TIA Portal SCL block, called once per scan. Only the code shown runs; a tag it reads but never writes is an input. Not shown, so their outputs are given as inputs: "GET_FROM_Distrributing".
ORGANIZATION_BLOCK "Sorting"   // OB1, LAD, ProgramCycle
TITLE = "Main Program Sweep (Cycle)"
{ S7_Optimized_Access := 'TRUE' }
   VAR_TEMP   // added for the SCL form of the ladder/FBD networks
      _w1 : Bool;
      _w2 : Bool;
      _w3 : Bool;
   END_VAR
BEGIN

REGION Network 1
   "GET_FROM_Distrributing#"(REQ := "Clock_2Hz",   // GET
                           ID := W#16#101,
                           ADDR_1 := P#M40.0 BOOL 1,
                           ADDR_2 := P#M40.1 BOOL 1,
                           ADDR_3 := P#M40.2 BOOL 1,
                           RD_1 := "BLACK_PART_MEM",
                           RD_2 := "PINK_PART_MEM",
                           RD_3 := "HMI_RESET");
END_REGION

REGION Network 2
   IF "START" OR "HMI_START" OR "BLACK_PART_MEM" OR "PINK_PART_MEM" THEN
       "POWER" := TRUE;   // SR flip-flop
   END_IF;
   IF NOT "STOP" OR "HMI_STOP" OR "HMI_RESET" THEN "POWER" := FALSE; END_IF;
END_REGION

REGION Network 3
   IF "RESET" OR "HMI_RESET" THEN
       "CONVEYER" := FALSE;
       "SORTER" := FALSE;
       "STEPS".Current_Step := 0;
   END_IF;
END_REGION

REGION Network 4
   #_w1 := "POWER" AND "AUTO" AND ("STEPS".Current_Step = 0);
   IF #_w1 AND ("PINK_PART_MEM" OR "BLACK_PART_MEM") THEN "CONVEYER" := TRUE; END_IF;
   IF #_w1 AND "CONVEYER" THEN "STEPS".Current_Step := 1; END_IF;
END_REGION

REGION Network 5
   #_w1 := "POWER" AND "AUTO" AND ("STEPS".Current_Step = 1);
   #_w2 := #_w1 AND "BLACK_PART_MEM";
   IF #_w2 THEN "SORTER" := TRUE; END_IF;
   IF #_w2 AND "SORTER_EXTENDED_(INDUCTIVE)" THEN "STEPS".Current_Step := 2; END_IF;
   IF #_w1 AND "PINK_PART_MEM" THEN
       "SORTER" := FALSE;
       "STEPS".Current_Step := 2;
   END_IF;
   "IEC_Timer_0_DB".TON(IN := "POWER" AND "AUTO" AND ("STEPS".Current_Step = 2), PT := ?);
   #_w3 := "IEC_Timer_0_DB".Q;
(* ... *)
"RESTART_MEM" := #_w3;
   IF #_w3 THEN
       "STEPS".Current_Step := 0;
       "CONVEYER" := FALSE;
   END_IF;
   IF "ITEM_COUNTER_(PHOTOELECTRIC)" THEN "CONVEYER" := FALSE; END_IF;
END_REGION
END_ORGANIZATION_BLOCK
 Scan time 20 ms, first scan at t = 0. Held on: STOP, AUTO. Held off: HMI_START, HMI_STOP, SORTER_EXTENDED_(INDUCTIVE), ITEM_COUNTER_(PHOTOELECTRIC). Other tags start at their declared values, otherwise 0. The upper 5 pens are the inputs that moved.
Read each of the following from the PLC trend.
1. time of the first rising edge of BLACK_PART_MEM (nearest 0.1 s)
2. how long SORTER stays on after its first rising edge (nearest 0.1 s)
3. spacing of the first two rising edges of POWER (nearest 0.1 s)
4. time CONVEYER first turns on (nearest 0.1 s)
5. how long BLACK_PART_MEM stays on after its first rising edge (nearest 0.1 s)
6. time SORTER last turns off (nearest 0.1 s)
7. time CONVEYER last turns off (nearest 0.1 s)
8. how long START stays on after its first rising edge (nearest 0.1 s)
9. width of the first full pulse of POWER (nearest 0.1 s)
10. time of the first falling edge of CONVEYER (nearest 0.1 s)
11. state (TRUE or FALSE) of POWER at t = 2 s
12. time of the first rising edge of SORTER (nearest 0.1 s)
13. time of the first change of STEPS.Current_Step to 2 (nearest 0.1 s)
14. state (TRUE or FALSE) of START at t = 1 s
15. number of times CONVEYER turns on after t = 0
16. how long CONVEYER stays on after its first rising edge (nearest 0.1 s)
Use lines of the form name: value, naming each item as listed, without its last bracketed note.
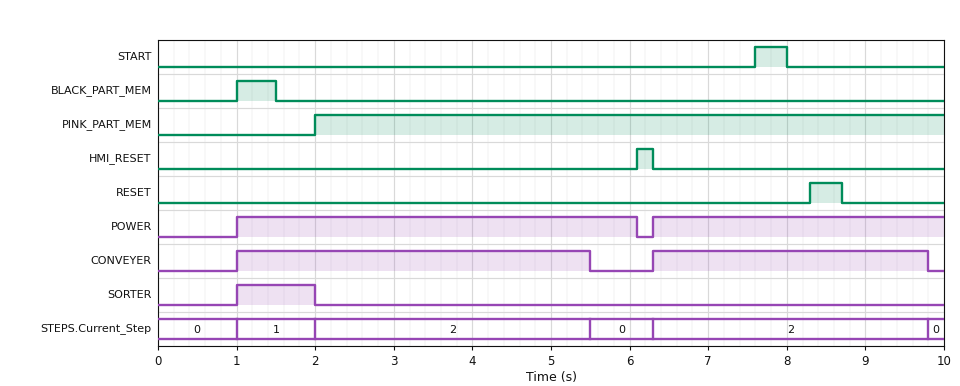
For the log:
time of the first rising edge of BLACK_PART_MEM: 1.0 s
how long SORTER stays on after its first rising edge: 1.0 s
spacing of the first two rising edges of POWER: 5.3 s
time CONVEYER first turns on: 1.0 s
how long BLACK_PART_MEM stays on after its first rising edge: 0.5 s
time SORTER last turns off: 2.0 s
time CONVEYER last turns off: 9.8 s
how long START stays on after its first rising edge: 0.4 s
width of the first full pulse of POWER: 5.1 s
time of the first falling edge of CONVEYER: 5.5 s
state (TRUE or FALSE) of POWER at t = 2 s: TRUE
time of the first rising edge of SORTER: 1.0 s
time of the first change of STEPS.Current_Step to 2: 2.0 s
state (TRUE or FALSE) of START at t = 1 s: FALSE
number of times CONVEYER turns on after t = 0: 2
how long CONVEYER stays on after its first rising edge: 4.5 s
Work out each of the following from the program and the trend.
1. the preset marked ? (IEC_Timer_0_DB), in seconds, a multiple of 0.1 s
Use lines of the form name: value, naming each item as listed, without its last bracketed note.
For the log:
the preset marked ? (IEC_Timer_0_DB), in seconds, a multiple of 0.1 s: 3.5 s
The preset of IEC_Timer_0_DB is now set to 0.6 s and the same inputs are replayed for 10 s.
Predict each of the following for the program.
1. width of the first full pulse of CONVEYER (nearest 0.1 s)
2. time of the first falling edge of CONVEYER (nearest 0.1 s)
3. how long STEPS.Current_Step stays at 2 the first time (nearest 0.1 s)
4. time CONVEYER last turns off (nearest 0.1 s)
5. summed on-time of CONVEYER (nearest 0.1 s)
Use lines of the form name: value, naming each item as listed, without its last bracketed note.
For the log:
width of the first full pulse of CONVEYER: 1.6 s
time of the first falling edge of CONVEYER: 2.6 s
how long STEPS.Current_Step stays at 2 the first time: 0.6 s
time CONVEYER last turns off: 6.9 s
summed on-time of CONVEYER: 2.2 s
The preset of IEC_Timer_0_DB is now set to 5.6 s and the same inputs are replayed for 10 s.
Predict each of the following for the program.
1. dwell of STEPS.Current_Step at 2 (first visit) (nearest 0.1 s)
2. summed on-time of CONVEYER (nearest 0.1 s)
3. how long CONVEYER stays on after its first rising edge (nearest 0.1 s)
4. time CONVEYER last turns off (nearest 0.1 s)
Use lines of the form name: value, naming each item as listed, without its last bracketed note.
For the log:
dwell of STEPS.Current_Step at 2 (first visit): 4.1 s
summed on-time of CONVEYER: 8.8 s
how long CONVEYER stays on after its first rising edge: 5.1 s
time CONVEYER last turns off: 6.1 s
